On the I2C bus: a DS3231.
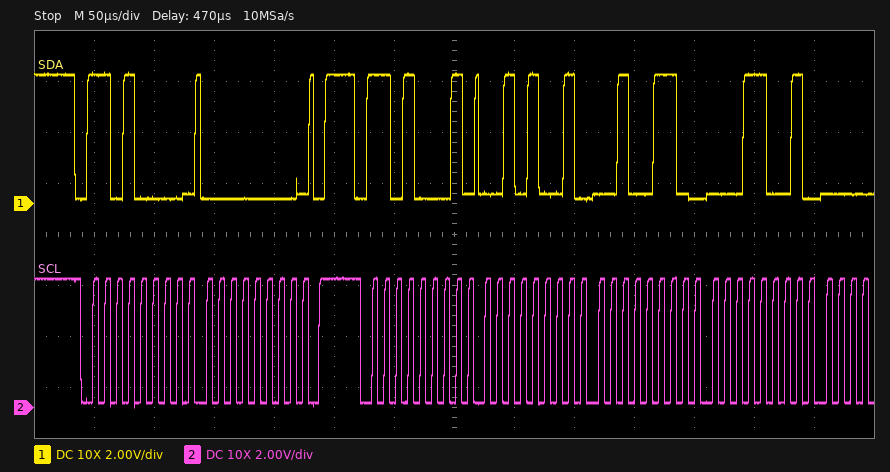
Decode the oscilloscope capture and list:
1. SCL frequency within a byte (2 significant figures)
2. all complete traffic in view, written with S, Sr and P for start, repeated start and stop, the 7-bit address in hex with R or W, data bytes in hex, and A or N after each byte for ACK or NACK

100 kHz
S 68W A 00 A P S 68R A 29 A 26 A 19 A
